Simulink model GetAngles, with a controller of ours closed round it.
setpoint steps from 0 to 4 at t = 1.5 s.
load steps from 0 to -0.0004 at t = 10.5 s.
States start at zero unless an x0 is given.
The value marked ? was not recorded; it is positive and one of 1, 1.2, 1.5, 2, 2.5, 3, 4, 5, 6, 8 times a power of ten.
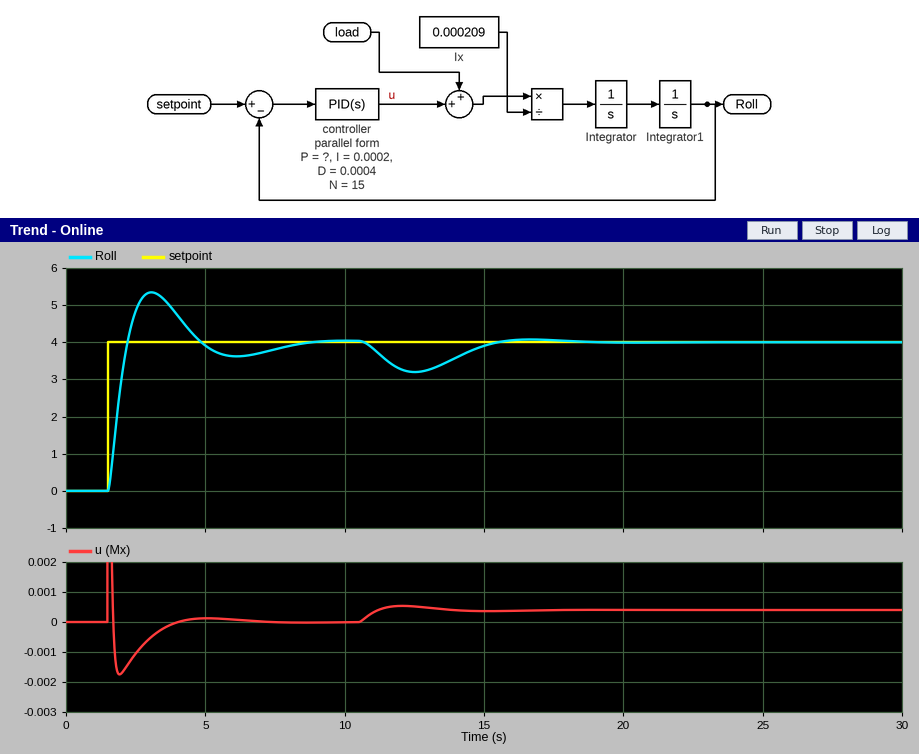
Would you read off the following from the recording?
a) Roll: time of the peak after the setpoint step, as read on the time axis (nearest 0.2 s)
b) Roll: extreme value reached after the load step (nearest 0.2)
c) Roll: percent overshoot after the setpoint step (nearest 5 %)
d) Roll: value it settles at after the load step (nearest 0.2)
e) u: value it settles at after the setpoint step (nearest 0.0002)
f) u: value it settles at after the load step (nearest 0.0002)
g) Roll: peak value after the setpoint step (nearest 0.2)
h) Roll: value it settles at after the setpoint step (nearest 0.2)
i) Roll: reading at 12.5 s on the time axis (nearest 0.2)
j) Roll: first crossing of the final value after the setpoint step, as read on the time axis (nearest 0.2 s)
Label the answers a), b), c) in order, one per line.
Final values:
a) 3.0 s
b) 3.2
c) 35 %
d) 4.0
e) 0.0000
f) 0.0004
g) 5.4
h) 4.0
i) 3.2
j) 2.2 s
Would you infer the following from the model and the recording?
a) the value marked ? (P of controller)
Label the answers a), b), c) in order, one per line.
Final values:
a) 0.0004
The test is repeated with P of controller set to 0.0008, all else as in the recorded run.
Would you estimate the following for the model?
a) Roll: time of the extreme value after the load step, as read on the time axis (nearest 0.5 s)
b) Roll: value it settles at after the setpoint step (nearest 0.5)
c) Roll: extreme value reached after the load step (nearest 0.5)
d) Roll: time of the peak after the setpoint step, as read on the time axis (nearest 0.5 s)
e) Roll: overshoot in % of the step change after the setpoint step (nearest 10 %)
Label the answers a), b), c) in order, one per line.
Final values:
a) 12.0 s
b) 4.0
c) 3.5
d) 2.5 s
e) 40 %
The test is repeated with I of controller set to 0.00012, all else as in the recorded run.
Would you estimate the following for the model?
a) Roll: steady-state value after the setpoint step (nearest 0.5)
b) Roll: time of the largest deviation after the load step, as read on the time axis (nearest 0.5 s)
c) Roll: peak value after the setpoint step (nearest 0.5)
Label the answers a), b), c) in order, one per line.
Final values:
a) 4.0
b) 12.5 s
c) 5.0
